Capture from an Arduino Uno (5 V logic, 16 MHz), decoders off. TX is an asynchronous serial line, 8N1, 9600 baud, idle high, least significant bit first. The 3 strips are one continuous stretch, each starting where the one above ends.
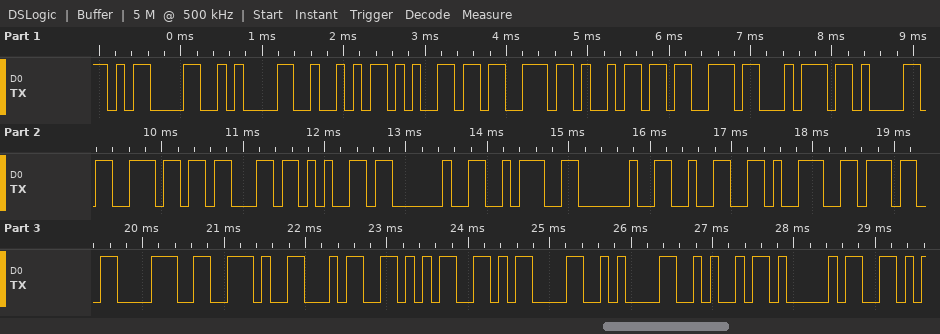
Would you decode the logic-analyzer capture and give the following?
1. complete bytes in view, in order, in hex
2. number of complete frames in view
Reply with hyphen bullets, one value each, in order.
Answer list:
- 0D 0A 52 65 73 69 73 74 61 6E 63 65 20 3A 20 32 39 37 38 2E 34 35 0D 0A 4A 41
- 26
